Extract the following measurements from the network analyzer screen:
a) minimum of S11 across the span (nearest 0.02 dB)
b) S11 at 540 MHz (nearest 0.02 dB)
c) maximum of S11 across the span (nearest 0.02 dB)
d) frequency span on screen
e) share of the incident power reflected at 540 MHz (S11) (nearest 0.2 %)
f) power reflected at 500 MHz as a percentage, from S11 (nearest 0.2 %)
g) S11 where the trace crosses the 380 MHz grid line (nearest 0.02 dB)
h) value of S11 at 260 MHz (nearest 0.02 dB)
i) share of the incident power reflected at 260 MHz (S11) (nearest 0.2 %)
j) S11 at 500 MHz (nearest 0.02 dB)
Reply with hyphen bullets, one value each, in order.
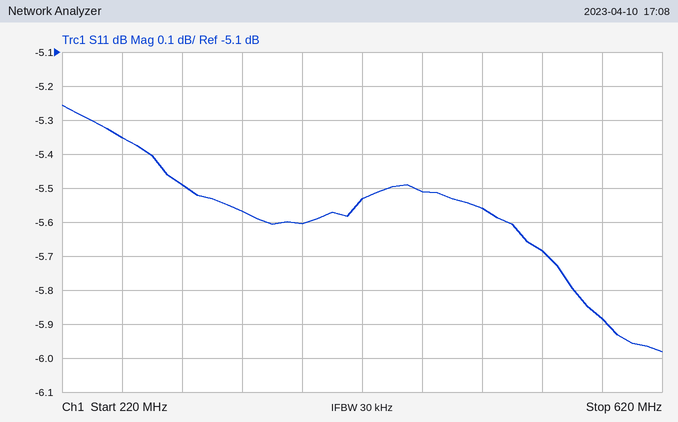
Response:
- -5.98 dB
- -5.68 dB
- -5.26 dB
- 400 MHz
- 27.0 %
- 27.8 %
- -5.60 dB
- -5.36 dB
- 29.2 %
- -5.56 dB
